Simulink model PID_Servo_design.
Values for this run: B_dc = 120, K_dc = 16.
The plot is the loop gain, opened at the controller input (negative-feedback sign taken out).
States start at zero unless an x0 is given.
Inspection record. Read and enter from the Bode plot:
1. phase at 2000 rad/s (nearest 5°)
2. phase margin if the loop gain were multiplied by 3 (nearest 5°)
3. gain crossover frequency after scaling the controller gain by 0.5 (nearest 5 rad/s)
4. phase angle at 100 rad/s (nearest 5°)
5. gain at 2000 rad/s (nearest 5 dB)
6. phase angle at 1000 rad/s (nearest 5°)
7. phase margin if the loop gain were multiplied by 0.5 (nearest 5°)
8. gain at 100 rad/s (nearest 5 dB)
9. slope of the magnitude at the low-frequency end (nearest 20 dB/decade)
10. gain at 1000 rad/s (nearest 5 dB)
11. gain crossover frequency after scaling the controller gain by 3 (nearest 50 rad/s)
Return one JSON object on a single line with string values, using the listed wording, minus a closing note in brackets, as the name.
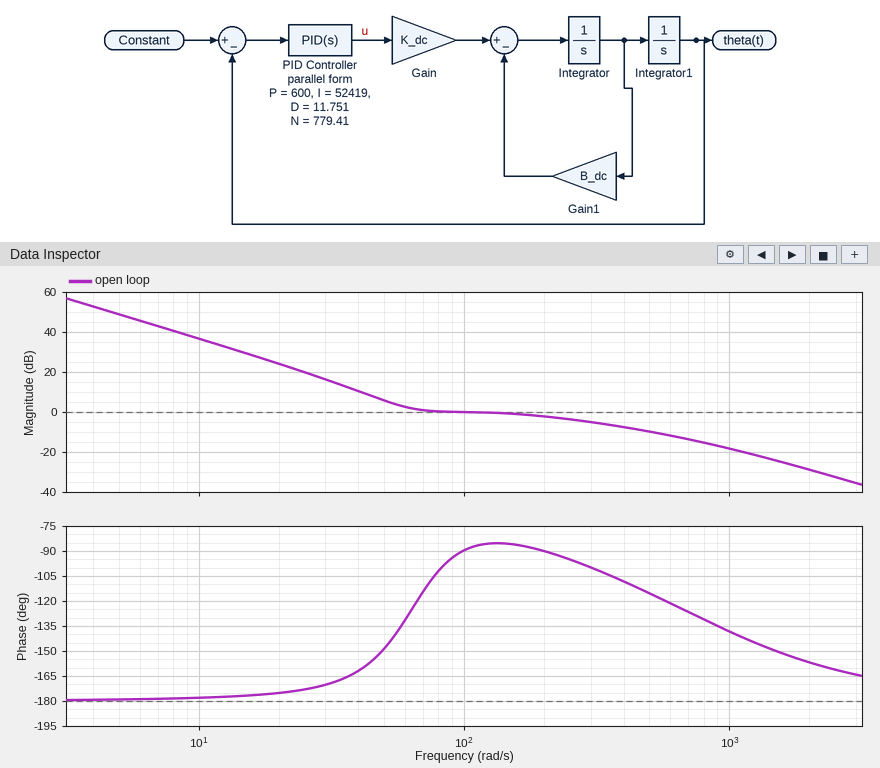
{"phase at 2000 rad/s": "-155°", "phase margin if the loop gain were multiplied by 3": "65°", "gain crossover frequency after scaling the controller gain by 0.5": "50 rad/s", "phase angle at 100 rad/s": "-90°", "gain at 2000 rad/s": "-30 dB", "phase angle at 1000 rad/s": "-140°", "phase margin if the loop gain were multiplied by 0.5": "30°", "gain at 100 rad/s": "0 dB", "slope of the magnitude at the low-frequency end": "-40 dB/decade", "gain at 1000 rad/s": "-20 dB", "gain crossover frequency after scaling the controller gain by 3": "500 rad/s"}
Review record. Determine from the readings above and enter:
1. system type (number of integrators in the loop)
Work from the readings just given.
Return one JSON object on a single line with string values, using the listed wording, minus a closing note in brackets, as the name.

{"system type": "2"}
